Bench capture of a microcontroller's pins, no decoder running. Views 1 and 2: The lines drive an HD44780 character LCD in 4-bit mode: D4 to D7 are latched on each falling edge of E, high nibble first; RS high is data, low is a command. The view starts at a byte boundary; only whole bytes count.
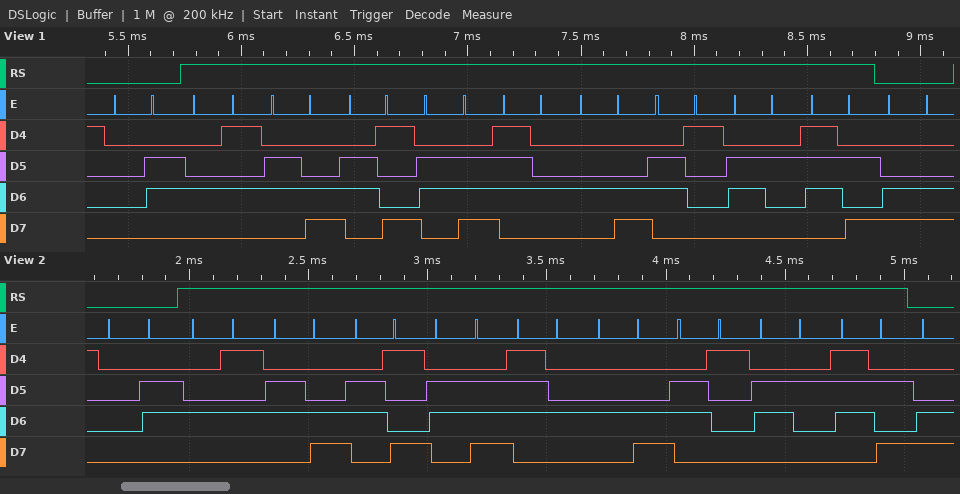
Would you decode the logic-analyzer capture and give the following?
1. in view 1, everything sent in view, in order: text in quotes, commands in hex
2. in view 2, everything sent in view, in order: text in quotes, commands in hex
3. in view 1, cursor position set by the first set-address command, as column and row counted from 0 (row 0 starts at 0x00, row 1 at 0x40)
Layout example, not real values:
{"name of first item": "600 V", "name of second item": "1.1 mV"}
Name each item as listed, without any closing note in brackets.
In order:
{"in view 1, everything sent in view, in order: text in quotes, commands in hex": "0x06 \"ElintLabz\" 0xCC", "in view 2, everything sent in view, in order: text in quotes, commands in hex": "0x06 \"ElintLabz\"", "in view 1, cursor position set by the first set-address command, as column and row counted from 0": "column 12, row 1"}
